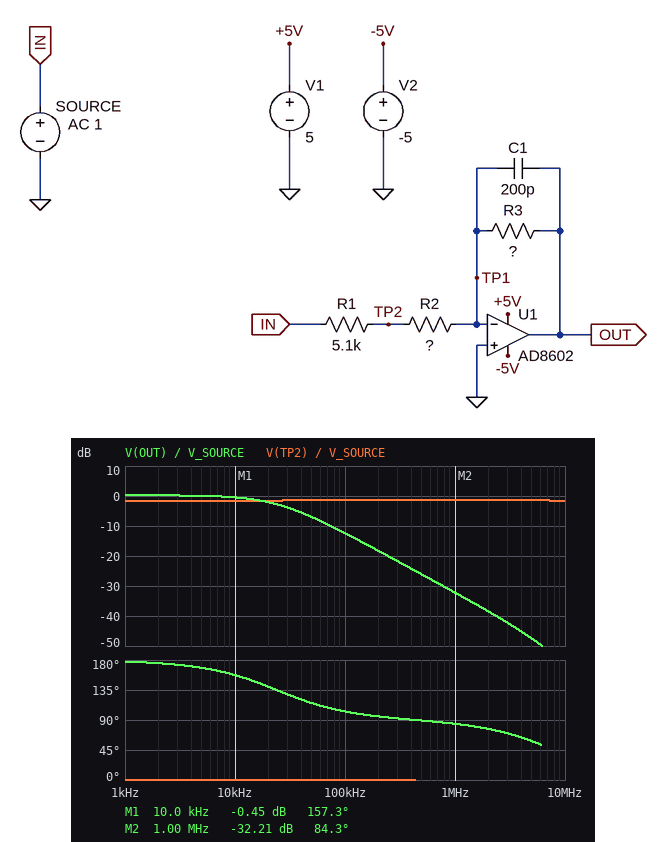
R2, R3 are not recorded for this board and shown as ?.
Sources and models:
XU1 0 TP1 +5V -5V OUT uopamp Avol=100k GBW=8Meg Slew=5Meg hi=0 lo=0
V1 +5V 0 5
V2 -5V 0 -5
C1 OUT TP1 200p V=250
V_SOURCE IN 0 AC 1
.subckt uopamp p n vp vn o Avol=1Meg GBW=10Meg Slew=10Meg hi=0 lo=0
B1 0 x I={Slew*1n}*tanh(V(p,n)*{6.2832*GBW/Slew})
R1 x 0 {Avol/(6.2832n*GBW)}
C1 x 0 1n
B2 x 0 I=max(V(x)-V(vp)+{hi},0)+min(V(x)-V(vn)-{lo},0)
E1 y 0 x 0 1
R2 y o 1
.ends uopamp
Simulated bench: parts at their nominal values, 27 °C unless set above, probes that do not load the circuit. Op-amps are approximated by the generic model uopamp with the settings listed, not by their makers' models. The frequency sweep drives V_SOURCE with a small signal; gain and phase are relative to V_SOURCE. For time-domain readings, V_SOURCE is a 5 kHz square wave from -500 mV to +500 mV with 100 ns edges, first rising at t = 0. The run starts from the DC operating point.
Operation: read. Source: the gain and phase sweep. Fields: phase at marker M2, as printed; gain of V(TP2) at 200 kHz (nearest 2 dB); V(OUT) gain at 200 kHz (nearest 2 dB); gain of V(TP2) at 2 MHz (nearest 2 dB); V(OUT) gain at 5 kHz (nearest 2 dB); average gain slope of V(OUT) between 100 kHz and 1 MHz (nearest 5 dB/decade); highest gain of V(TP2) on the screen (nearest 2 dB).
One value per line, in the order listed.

84.3 deg
-2 dB
-18 dB
-2 dB
0 dB
-20 dB/decade
-2 dB
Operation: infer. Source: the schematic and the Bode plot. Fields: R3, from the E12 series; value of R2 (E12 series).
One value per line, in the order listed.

33 kΩ
27 kΩ
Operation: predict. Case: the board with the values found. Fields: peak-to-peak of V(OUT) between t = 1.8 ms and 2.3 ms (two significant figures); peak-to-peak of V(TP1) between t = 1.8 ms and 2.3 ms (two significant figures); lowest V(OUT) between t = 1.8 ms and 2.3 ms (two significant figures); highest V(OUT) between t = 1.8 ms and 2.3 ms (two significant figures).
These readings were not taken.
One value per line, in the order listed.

1.0 V
6.1 mV
-510 mV
510 mV
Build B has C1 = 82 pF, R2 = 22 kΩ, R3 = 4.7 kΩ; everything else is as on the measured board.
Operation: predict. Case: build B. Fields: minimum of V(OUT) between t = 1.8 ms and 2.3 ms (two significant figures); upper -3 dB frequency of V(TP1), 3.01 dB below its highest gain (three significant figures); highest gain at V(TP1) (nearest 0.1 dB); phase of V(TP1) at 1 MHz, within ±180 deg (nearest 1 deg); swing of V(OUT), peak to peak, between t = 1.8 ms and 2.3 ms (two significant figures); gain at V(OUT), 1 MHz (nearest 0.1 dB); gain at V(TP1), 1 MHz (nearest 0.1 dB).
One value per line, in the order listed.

-87 mV
8.86 MHz
-41.5 dB
15 deg
170 mV
-23.7 dB
-41.8 dB
